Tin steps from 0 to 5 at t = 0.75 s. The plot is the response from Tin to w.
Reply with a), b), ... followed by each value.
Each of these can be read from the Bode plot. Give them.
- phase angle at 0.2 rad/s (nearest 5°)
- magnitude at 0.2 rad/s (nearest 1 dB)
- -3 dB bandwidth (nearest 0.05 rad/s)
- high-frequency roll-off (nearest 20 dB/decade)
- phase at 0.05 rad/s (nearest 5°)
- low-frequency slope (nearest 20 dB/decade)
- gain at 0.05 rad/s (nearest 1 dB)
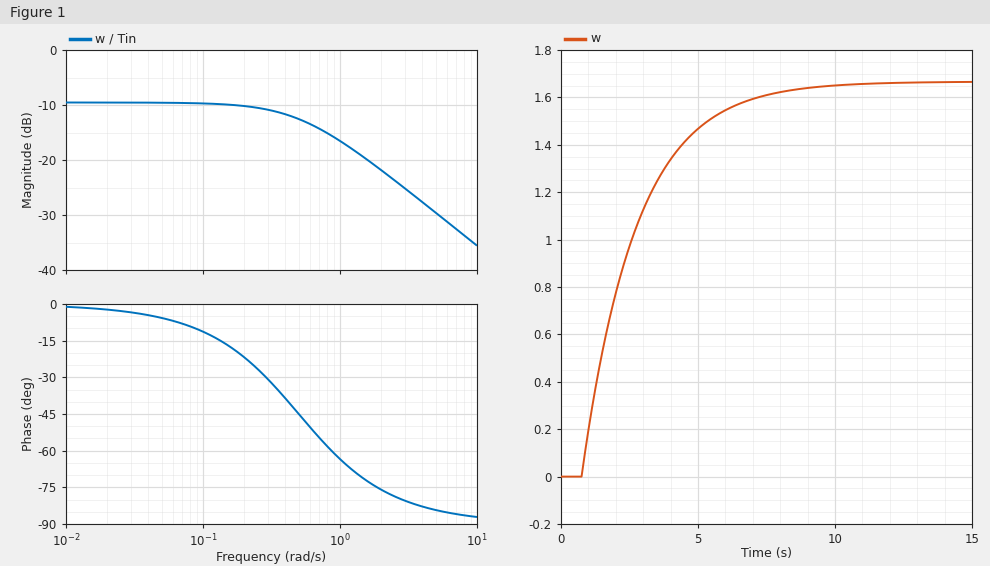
a) -20°
b) -10 dB
c) 0.50 rad/s
d) -20 dB/decade
e) -5°
f) 0 dB/decade
g) -10 dB
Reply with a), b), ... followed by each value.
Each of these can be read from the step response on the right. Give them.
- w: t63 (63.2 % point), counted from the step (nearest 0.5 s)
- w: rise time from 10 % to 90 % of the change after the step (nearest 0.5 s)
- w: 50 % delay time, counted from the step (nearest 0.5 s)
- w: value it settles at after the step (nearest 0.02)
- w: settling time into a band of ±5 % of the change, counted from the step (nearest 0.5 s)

a) 2.0 s
b) 4.5 s
c) 1.5 s
d) 1.66
e) 6.0 s
